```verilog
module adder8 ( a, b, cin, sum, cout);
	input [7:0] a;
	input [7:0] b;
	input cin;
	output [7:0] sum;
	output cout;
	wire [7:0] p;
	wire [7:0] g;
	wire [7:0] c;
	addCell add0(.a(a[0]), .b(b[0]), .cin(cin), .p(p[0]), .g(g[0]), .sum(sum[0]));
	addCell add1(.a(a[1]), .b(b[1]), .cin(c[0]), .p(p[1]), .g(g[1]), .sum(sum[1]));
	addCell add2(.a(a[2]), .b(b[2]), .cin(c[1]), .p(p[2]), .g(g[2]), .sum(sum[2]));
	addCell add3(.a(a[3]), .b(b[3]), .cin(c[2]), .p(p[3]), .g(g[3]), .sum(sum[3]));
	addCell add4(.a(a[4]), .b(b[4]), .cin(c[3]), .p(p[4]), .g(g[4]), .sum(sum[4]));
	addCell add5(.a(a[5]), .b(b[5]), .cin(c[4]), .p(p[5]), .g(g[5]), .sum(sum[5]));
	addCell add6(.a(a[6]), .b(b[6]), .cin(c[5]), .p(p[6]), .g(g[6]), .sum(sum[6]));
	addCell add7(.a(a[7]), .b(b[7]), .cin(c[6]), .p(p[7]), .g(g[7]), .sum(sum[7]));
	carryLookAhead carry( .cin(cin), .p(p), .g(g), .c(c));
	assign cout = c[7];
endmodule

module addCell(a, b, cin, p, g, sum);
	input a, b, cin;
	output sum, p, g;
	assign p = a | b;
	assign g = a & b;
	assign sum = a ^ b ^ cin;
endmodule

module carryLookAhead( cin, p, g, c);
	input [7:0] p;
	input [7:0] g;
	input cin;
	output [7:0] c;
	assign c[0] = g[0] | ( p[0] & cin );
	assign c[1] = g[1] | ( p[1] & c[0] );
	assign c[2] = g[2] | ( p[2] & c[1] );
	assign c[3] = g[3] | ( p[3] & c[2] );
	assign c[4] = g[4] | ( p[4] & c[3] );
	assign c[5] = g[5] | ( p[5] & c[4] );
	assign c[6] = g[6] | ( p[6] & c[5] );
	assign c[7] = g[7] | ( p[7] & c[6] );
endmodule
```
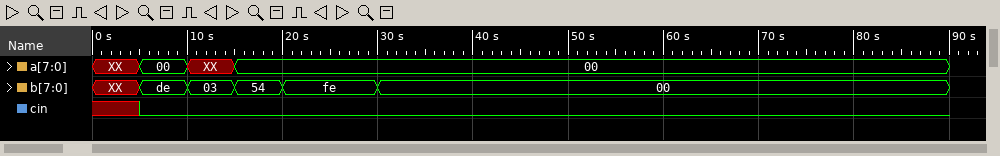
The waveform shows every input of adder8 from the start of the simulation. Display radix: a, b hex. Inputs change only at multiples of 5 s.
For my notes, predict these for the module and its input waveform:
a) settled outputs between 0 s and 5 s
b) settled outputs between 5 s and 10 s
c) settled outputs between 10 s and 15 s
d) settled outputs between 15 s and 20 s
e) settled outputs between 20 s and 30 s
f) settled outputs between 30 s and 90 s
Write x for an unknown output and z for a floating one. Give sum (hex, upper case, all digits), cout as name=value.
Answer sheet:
sum=x, cout=x
sum=DE, cout=0
sum=x, cout=x
sum=54, cout=0
sum=FE, cout=0
sum=00, cout=0
